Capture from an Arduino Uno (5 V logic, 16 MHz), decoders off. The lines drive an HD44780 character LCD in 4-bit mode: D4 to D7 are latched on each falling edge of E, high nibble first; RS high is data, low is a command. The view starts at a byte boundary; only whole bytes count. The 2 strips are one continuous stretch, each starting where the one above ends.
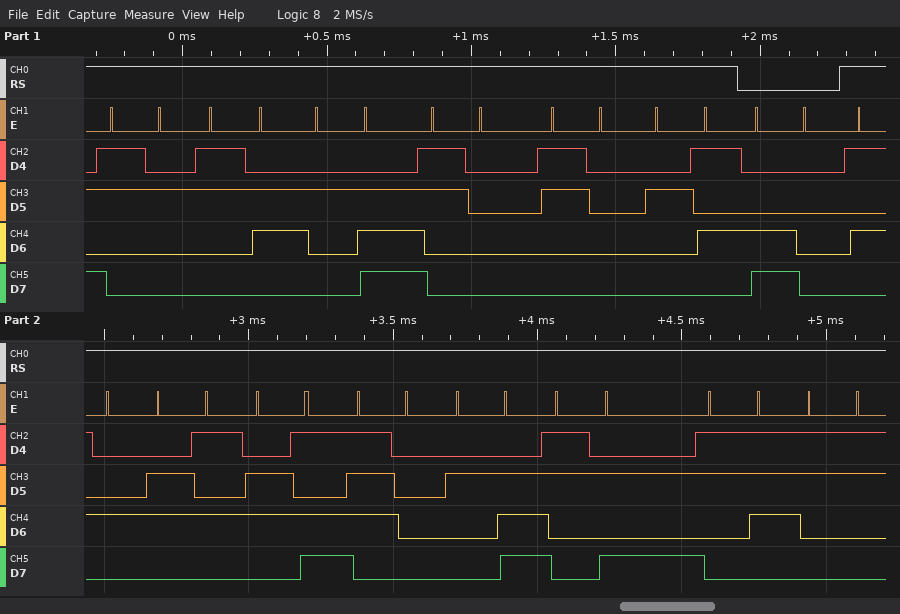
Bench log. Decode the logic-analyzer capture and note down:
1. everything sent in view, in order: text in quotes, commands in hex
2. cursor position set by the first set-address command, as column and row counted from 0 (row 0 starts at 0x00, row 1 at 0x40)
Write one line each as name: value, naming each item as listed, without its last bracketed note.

everything sent in view, in order: text in quotes, commands in hex: "26.00%" 0xC0 "Temp.:73"
cursor position set by the first set-address command, as column and row counted from 0: column 0, row 1
